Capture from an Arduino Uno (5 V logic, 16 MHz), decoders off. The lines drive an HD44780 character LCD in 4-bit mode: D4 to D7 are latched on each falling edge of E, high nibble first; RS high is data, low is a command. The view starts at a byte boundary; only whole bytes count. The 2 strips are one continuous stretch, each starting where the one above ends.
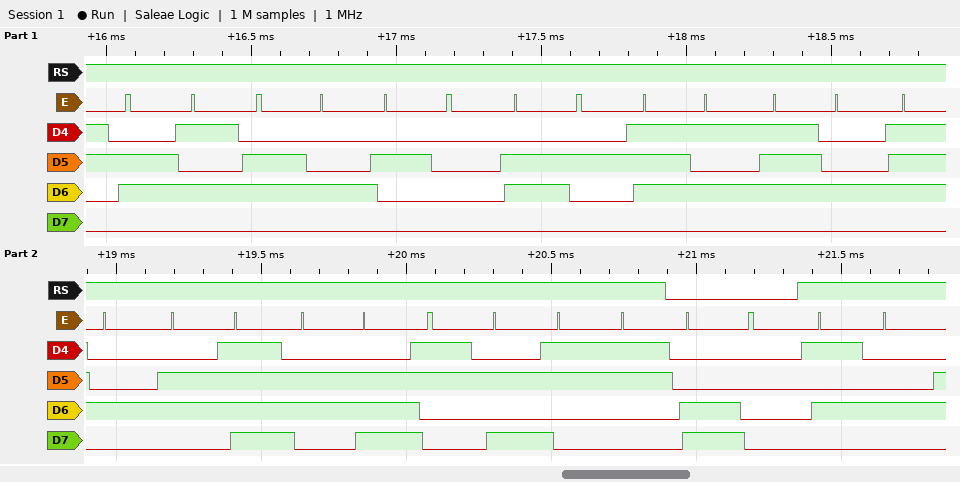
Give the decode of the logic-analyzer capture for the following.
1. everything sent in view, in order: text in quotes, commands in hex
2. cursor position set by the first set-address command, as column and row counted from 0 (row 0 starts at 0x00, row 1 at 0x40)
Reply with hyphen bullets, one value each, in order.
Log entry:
- "ed button:3" 0xC0 "T"
- column 0, row 1
